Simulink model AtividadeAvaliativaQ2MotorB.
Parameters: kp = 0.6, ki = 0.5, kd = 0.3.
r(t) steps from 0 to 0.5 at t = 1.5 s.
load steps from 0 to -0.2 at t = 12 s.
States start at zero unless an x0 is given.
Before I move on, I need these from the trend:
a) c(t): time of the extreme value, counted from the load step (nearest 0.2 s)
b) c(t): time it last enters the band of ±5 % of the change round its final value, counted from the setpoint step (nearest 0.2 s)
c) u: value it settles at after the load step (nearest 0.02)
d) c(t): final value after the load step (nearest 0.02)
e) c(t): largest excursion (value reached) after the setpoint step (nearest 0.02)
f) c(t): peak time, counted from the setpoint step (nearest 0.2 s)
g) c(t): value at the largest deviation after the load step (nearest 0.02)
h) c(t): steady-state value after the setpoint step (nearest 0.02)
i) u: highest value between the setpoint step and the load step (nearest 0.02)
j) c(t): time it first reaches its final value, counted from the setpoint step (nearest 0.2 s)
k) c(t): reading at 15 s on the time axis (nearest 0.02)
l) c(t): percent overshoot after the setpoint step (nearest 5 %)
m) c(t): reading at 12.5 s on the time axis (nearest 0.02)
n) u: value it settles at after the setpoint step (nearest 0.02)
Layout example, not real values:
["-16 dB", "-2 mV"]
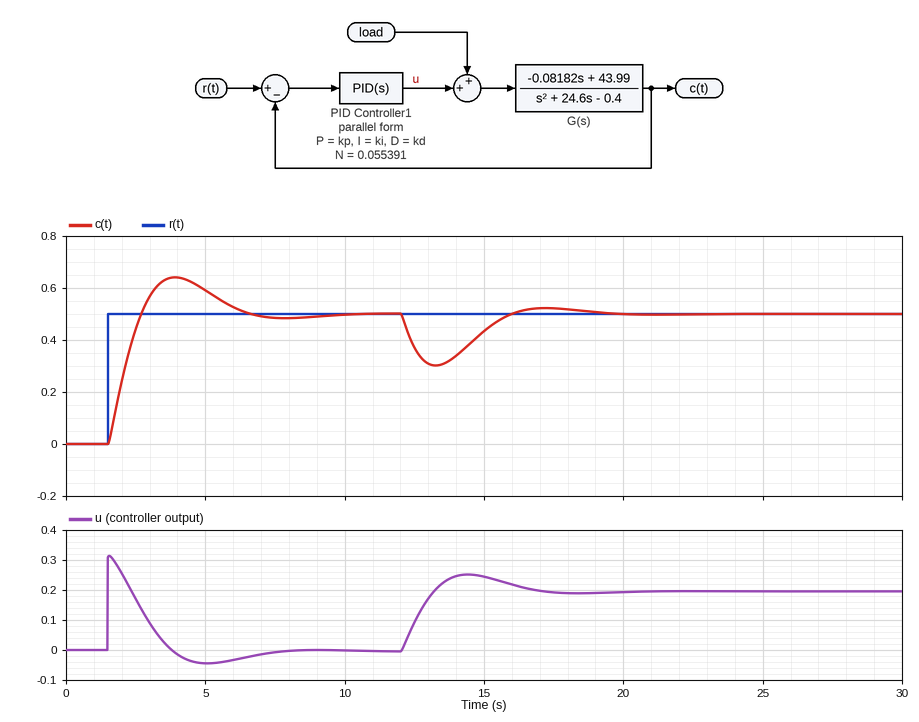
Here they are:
["1.2 s", "4.6 s", "0.20", "0.50", "0.64", "2.4 s", "0.30", "0.50", "0.32", "1.2 s", "0.44", "30 %", "0.38", "0.00"]
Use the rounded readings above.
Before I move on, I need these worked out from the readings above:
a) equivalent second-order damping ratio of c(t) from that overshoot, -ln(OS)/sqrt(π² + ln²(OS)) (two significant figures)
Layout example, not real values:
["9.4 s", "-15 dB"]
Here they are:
["0.36"]
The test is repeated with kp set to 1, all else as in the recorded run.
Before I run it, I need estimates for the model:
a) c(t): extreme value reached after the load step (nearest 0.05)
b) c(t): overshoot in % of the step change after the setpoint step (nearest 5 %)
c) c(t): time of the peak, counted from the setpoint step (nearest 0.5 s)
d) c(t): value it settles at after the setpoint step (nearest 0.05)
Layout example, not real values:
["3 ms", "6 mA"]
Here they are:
["0.35", "15 %", "2.0 s", "0.50"]
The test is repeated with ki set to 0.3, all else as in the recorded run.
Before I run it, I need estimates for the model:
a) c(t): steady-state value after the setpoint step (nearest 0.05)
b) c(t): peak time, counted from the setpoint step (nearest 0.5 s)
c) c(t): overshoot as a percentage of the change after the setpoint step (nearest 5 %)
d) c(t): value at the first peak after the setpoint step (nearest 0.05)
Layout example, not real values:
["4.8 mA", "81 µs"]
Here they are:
["0.50", "3.0 s", "20 %", "0.60"]
